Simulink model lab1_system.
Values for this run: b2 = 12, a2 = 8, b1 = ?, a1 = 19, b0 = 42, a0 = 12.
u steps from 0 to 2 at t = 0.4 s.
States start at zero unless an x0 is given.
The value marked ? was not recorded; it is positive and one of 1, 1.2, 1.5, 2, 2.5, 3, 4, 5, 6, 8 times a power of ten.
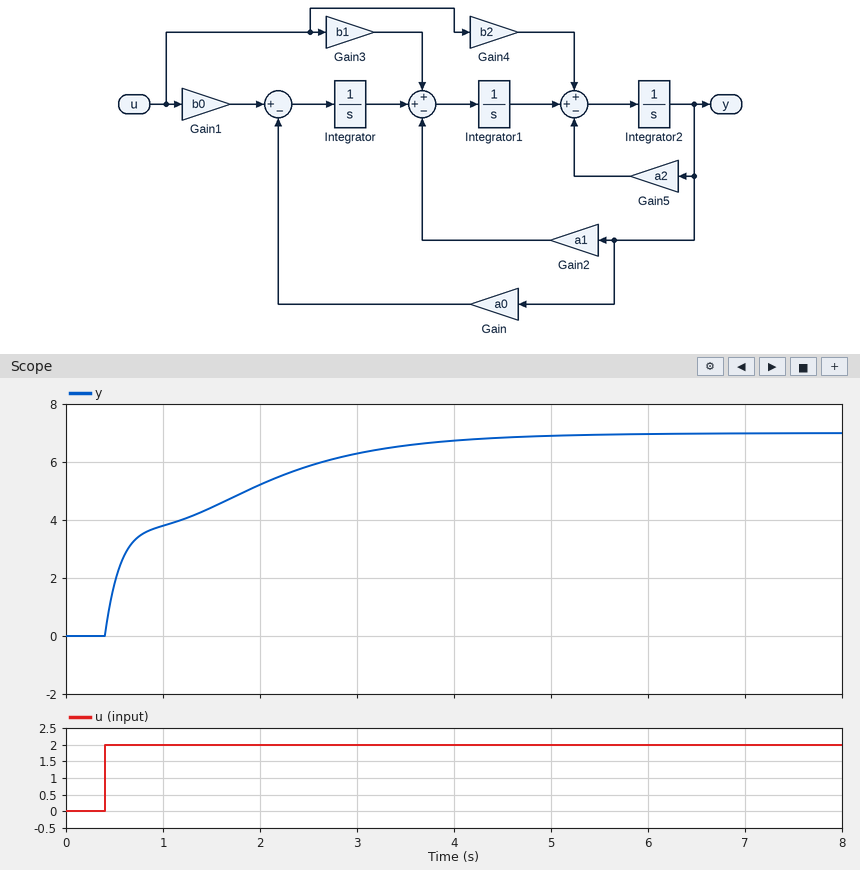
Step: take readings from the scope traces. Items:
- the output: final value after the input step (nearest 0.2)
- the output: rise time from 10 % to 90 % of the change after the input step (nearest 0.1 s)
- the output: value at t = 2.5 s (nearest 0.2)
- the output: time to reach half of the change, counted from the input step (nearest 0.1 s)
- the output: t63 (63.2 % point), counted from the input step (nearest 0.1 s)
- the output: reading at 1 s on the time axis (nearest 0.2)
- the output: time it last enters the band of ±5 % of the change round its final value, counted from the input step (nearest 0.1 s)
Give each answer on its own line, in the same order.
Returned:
7.0
2.6 s
5.8
0.4 s
1.1 s
3.8
3.3 s
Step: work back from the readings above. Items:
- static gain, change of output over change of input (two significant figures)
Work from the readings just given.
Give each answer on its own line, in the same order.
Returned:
3.5
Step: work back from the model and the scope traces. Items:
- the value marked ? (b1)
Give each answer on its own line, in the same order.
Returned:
25
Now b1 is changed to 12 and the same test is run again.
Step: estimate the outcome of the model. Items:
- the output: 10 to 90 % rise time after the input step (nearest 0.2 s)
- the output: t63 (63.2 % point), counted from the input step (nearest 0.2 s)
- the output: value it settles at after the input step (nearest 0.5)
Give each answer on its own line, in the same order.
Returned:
3.0 s
1.6 s
7.0
